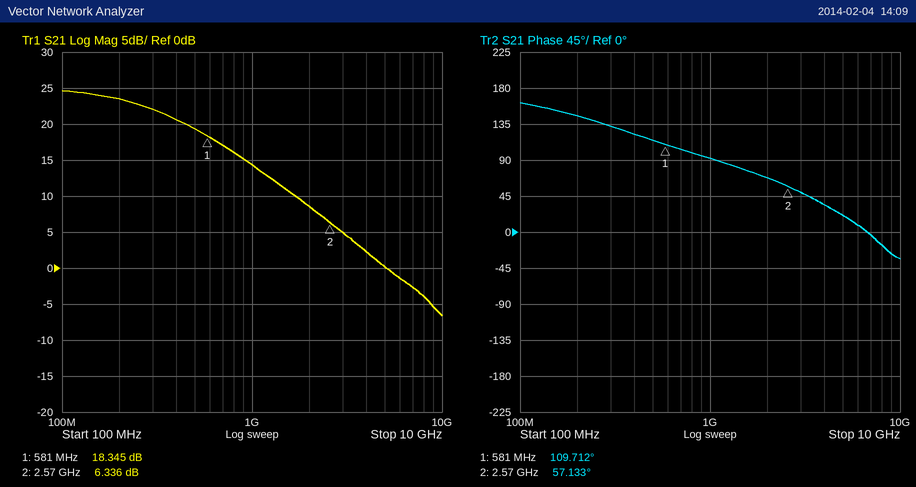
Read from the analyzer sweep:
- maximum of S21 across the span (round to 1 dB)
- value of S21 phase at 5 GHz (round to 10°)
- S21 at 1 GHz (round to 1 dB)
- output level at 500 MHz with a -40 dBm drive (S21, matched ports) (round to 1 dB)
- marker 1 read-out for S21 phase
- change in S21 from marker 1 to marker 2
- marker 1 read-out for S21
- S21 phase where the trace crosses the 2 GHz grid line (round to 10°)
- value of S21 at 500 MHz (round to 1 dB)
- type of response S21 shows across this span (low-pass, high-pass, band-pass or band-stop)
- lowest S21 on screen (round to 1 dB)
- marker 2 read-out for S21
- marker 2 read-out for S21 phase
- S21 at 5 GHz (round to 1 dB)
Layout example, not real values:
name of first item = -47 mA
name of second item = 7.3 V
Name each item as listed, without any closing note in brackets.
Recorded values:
maximum of S21 across the span = 25 dB
value of S21 phase at 5 GHz = 20°
S21 at 1 GHz = 14 dB
output level at 500 MHz with a -40 dBm drive (S21, matched ports) = -21 dBm
marker 1 read-out for S21 phase = 109.712°
change in S21 from marker 1 to marker 2 = -12.009 dB
marker 1 read-out for S21 = 18.345 dB
S21 phase where the trace crosses the 2 GHz grid line = 70°
value of S21 at 500 MHz = 19 dB
type of response S21 shows across this span = low-pass
lowest S21 on screen = -7 dB
marker 2 read-out for S21 = 6.336 dB
marker 2 read-out for S21 phase = 57.133°
S21 at 5 GHz = 0 dB
